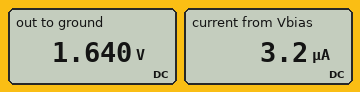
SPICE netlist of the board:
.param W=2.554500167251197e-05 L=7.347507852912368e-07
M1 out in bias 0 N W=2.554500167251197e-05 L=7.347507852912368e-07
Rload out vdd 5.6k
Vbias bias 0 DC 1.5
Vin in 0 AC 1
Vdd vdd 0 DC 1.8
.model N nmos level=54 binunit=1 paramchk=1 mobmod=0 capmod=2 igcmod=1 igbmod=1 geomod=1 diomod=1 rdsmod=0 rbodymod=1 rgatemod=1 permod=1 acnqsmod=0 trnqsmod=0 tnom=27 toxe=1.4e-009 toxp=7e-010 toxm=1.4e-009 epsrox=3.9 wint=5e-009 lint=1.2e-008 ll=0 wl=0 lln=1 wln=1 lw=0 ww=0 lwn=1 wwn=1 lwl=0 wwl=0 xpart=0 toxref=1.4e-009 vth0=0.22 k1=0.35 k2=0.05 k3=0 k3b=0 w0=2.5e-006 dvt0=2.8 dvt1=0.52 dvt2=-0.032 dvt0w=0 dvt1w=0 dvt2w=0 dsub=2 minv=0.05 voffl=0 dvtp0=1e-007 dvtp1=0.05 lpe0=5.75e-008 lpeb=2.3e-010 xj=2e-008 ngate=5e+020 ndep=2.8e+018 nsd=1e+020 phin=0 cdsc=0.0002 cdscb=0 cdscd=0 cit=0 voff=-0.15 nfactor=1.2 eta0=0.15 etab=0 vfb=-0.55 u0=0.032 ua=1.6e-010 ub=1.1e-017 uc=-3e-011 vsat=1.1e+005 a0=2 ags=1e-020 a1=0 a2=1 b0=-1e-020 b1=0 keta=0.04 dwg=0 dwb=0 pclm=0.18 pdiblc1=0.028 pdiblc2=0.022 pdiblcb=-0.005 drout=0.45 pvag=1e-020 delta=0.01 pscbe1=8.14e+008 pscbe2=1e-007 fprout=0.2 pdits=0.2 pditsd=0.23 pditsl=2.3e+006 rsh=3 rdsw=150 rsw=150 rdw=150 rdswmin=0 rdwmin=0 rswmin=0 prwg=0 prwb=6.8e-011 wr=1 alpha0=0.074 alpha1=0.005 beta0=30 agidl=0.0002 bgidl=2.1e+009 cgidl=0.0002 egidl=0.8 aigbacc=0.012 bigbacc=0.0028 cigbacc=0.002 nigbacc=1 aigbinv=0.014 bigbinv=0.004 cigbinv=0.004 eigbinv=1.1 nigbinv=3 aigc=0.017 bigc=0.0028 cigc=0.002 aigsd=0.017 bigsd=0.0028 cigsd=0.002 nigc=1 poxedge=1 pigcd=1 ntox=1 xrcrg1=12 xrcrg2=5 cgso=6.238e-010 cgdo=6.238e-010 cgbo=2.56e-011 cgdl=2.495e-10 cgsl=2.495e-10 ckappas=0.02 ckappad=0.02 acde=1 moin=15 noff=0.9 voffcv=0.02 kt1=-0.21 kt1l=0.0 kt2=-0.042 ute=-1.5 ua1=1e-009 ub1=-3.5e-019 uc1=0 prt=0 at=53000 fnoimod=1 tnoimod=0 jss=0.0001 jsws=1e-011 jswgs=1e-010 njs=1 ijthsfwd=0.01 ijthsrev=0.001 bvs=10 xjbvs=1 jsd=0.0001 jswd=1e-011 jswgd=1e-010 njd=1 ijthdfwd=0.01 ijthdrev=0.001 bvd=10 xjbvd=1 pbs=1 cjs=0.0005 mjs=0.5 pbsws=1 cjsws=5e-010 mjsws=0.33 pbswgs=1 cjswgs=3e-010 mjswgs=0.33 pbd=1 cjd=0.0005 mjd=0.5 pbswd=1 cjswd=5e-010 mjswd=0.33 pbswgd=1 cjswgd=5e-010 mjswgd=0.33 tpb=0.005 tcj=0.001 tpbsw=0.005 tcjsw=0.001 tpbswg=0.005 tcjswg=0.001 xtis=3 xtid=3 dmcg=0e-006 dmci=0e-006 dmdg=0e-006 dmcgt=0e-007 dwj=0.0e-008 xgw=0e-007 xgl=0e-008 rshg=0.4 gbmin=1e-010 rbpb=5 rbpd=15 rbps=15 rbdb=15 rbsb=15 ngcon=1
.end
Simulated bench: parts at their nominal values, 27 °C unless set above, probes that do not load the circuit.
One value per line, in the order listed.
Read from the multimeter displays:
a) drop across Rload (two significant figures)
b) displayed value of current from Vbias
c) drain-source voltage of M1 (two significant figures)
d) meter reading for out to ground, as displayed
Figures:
160 mV
3.2 µA
140 mV
1.640 V
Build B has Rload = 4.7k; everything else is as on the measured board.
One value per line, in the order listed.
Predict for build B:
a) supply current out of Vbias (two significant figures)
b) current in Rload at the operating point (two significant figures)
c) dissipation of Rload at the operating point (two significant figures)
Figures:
3.2 µA
32 µA
4.9 µW
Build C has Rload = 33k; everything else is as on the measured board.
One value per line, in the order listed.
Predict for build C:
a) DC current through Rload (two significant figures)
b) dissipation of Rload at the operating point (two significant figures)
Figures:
7.6 µA
1.9 µW
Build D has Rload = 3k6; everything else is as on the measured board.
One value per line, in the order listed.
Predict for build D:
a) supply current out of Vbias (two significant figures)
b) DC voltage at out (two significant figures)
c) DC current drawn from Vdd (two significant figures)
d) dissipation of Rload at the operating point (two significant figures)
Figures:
3.2 µA
1.7 V
38 µA
5.3 µW
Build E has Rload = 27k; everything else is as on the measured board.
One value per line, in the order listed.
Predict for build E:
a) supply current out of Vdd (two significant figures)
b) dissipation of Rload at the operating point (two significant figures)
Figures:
8.9 µA
2.1 µW
